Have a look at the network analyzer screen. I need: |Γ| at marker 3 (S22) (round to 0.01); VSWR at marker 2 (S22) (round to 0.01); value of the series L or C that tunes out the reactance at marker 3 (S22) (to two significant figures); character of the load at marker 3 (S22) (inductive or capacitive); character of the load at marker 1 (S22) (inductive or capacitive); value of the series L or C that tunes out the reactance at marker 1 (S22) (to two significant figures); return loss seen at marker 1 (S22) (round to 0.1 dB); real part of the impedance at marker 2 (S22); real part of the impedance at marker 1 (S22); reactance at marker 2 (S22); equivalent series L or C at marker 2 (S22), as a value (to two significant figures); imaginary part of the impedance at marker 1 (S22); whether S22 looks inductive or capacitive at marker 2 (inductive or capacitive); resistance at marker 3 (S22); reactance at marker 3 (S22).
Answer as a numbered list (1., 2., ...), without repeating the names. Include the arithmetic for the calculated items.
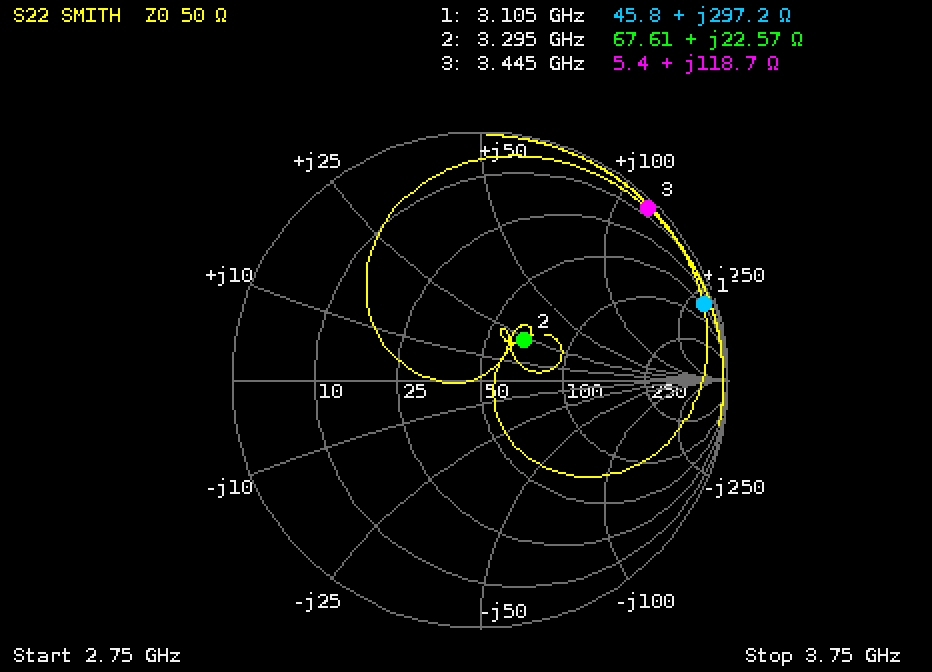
1. 0.97
2. 1.63
3. C = 1/(2π × 3.445 GHz × 118.7 Ω) ≈ 389 fF, so 390 fF to two significant figures
4. inductive
5. inductive
6. C = 1/(2π × 3.105 GHz × 297.2 Ω) ≈ 172 fF, so 170 fF to two significant figures
7. 0.4 dB
8. 67.61 Ω
9. 45.8 Ω
10. +22.57 Ω
11. L = 22.57 Ω/(2π × 3.295 GHz) ≈ 1.1 nH
12. +297.2 Ω
13. inductive
14. 5.4 Ω
15. +118.7 Ω
